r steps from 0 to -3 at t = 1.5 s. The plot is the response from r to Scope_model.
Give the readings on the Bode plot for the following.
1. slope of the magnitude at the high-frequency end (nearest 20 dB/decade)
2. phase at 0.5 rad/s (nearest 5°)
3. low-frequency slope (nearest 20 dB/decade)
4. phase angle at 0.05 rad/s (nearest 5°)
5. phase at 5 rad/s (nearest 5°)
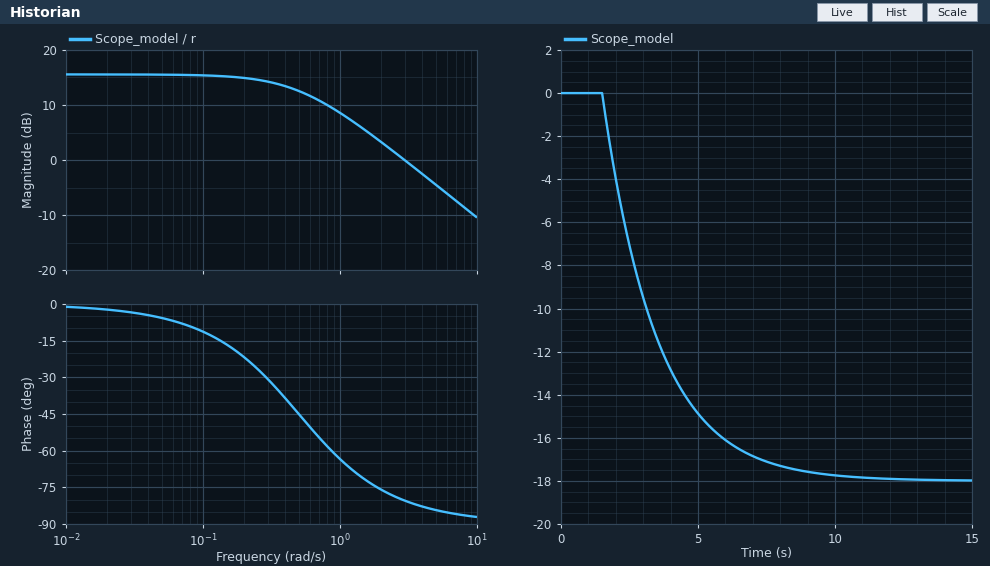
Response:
-20 dB/decade
-45°
0 dB/decade
-5°
-85°
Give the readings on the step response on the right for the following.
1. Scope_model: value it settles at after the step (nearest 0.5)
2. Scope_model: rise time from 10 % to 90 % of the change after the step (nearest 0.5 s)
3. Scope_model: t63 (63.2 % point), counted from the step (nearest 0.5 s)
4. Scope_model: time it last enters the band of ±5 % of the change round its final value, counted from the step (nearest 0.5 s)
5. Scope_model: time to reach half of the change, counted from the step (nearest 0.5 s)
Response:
-18.0
4.5 s
2.0 s
6.0 s
1.5 s
